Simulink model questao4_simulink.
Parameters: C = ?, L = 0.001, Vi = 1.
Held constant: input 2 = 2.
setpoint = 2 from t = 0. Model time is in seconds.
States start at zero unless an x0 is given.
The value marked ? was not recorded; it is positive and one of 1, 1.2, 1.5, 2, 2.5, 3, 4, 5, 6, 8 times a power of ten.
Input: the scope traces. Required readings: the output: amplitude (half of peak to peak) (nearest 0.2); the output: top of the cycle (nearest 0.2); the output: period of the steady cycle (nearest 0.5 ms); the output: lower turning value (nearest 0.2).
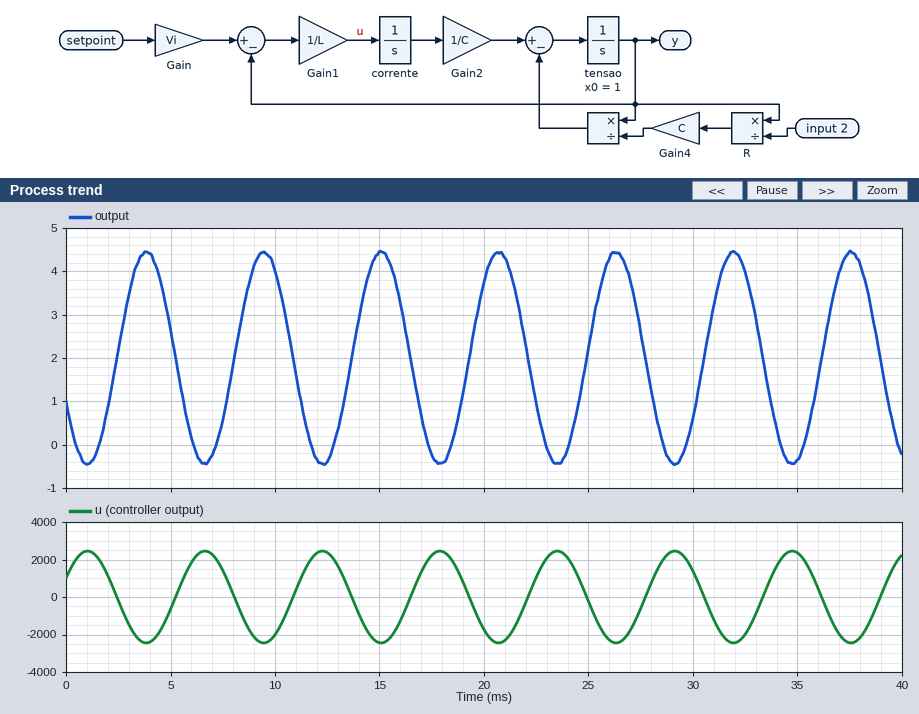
2.4
4.4
5.5 ms
-0.4
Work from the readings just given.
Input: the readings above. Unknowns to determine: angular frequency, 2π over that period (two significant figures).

1.1 rad/ms
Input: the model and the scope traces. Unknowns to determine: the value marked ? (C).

0.0008
